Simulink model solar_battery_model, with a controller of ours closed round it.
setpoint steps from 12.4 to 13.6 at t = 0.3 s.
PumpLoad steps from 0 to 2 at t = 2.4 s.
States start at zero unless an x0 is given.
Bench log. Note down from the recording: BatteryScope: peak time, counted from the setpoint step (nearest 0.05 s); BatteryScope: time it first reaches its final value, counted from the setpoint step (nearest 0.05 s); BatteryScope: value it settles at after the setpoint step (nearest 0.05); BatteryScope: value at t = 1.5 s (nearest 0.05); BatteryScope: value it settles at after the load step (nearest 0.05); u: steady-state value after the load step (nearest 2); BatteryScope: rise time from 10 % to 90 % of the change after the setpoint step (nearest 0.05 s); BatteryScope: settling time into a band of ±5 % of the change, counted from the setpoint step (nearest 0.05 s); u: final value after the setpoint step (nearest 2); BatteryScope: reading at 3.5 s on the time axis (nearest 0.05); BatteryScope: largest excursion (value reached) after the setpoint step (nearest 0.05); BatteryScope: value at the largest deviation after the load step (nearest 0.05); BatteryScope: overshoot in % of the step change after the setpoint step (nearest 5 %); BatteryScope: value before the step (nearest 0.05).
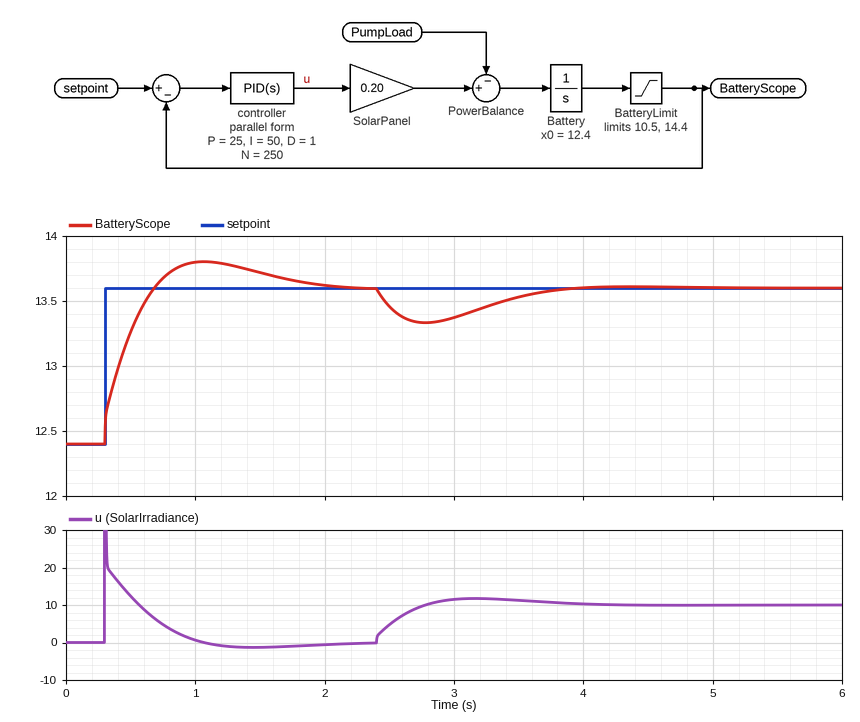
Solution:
0.75 s
0.40 s
13.60
13.70
13.60
10
0.30 s
1.45 s
0
13.55
13.80
13.35
15 %
12.40
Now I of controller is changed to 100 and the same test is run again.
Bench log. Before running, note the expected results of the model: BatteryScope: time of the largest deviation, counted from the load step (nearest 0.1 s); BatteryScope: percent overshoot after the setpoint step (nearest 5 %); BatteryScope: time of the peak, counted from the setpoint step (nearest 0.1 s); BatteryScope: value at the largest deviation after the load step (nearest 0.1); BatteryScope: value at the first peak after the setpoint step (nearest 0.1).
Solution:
0.3 s
25 %
0.6 s
13.4
13.9
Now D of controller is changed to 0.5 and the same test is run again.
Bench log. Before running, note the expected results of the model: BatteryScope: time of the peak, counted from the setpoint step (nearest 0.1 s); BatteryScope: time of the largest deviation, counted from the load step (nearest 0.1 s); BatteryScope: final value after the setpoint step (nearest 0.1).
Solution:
0.7 s
0.4 s
13.6
